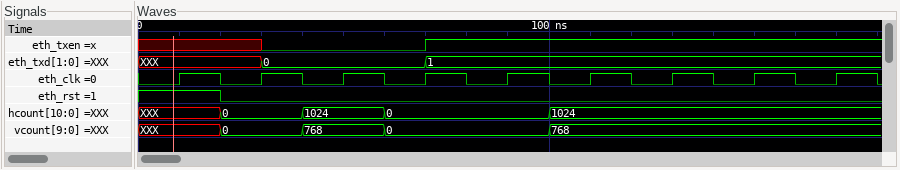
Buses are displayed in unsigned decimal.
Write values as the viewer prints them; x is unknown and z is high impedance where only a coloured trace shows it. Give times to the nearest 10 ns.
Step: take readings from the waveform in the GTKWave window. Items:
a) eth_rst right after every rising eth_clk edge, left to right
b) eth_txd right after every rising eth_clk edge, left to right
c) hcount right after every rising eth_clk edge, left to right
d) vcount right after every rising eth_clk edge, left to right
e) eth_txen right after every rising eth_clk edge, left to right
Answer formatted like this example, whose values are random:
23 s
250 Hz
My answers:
1 0 0 0 0 0 0 0 0
XXX, 0, 0, 1, 1, 1, 1, 1, 1
XXX, 0, 1024, 0, 0, 1024, 1024, 1024, 1024
XXX, 0, 768, 0, 0, 768, 768, 768, 768
x 0 0 1 1 1 1 1 1
